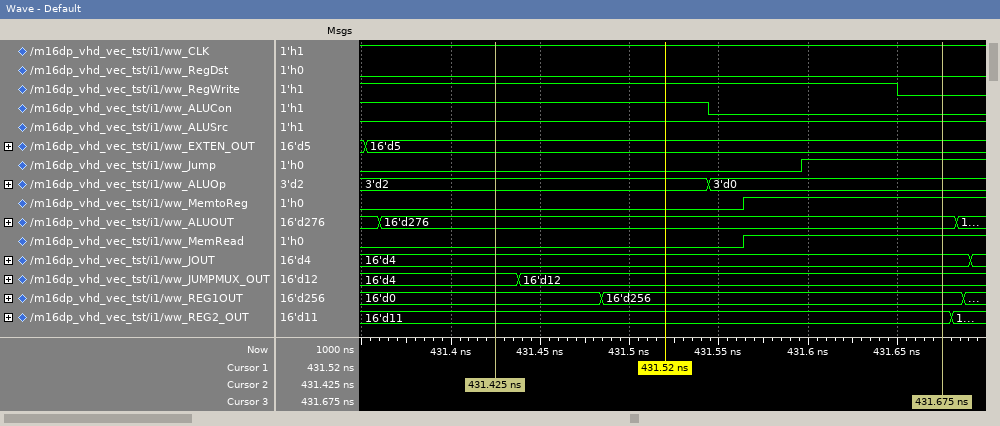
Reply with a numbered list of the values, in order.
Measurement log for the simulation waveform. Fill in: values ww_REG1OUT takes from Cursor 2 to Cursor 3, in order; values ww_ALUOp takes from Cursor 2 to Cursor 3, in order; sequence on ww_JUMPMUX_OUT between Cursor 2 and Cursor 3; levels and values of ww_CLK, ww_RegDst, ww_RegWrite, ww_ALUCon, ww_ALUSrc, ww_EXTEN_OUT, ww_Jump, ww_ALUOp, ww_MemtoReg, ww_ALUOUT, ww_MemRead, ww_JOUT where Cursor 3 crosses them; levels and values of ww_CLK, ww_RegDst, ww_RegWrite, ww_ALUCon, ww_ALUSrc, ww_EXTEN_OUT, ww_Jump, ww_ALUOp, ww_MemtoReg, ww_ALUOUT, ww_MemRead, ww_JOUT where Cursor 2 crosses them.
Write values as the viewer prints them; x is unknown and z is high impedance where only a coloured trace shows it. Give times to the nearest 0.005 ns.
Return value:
1. 16'd0, 16'd256
2. 3'd2, 3'd0
3. 16'd4, 16'd12
4. ww_CLK=1, ww_RegDst=0, ww_RegWrite=0, ww_ALUCon=0, ww_ALUSrc=1, ww_EXTEN_OUT=16'd5, ww_Jump=1, ww_ALUOp=3'd0, ww_MemtoReg=1, ww_ALUOUT=16'd276, ww_MemRead=1, ww_JOUT=16'd4
5. ww_CLK=1, ww_RegDst=0, ww_RegWrite=1, ww_ALUCon=1, ww_ALUSrc=1, ww_EXTEN_OUT=16'd5, ww_Jump=0, ww_ALUOp=3'd2, ww_MemtoReg=0, ww_ALUOUT=16'd276, ww_MemRead=0, ww_JOUT=16'd4
